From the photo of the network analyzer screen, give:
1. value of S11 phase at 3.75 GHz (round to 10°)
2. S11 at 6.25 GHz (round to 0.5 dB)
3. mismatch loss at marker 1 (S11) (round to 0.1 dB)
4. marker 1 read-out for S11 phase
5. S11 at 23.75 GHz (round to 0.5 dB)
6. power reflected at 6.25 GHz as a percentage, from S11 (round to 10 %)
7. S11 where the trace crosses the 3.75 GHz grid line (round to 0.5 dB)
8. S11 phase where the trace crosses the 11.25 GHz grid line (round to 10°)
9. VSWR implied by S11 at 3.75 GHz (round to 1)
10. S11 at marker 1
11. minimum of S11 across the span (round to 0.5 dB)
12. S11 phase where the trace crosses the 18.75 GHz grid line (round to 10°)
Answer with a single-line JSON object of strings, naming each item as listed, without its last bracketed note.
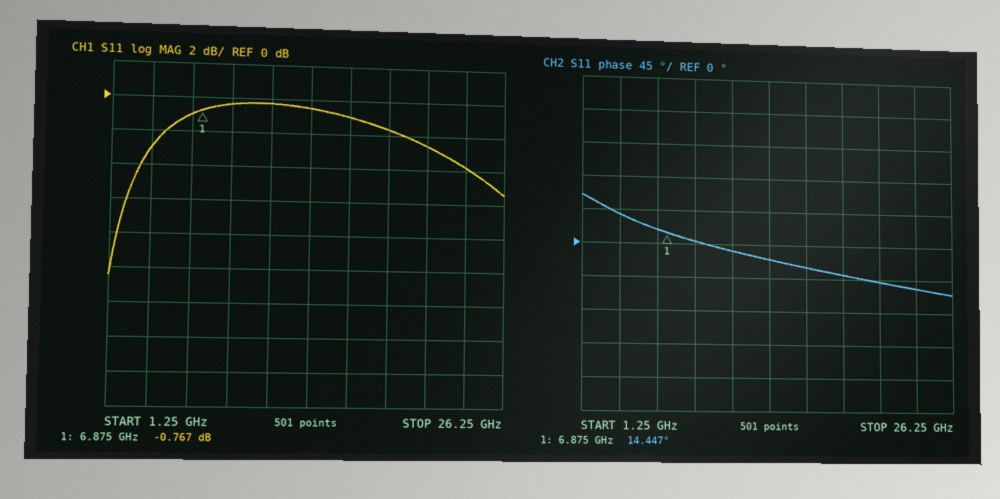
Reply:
{"value of S11 phase at 3.75 GHz": "40°", "S11 at 6.25 GHz": "-1.0 dB", "mismatch loss at marker 1 (S11)": "7.9 dB", "marker 1 read-out for S11 phase": "14.447°", "S11 at 23.75 GHz": "-4.0 dB", "power reflected at 6.25 GHz as a percentage, from S11": "80 %", "S11 where the trace crosses the 3.75 GHz grid line": "-3.0 dB", "S11 phase where the trace crosses the 11.25 GHz grid line": "-10°", "VSWR implied by S11 at 3.75 GHz": "6", "S11 at marker 1": "-0.767 dB", "minimum of S11 across the span": "-10.5 dB", "S11 phase where the trace crosses the 18.75 GHz grid line": "-40°"}
